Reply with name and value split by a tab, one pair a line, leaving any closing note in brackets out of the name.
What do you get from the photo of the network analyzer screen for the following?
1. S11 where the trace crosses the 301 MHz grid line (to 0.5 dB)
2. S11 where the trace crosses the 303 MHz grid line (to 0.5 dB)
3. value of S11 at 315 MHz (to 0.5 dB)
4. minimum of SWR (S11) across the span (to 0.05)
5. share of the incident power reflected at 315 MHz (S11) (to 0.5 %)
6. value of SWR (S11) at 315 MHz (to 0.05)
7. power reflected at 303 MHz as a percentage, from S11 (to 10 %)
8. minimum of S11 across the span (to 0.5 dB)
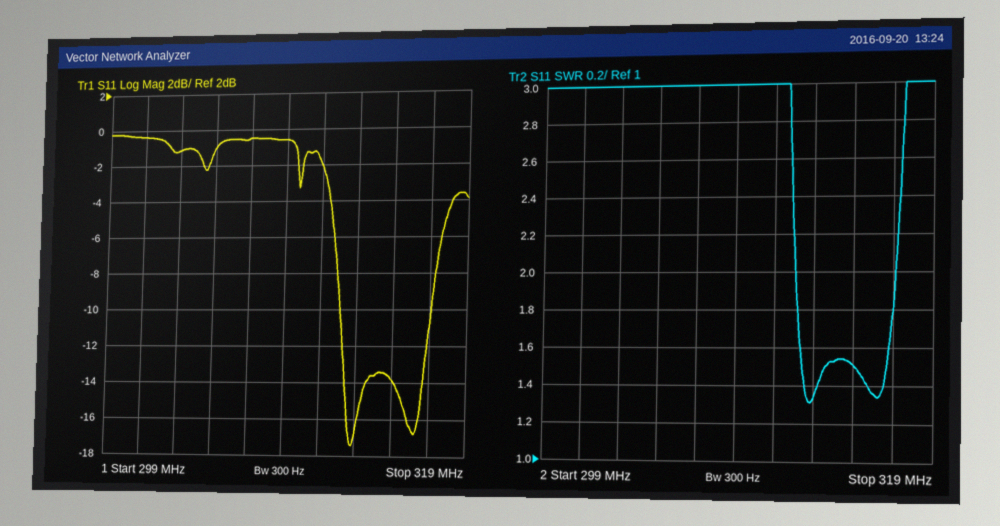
S11 where the trace crosses the 301 MHz grid line	-0.5 dB
S11 where the trace crosses the 303 MHz grid line	-1.0 dB
value of S11 at 315 MHz	-14.0 dB
minimum of SWR (S11) across the span	1.30
share of the incident power reflected at 315 MHz (S11)	4.0 %
value of SWR (S11) at 315 MHz	1.50
power reflected at 303 MHz as a percentage, from S11	80 %
minimum of S11 across the span	-17.5 dB
